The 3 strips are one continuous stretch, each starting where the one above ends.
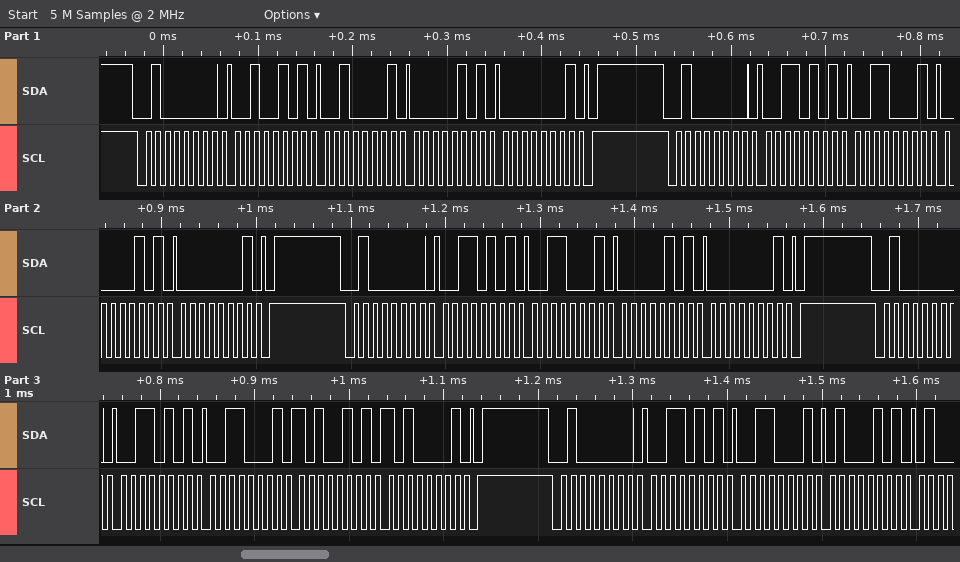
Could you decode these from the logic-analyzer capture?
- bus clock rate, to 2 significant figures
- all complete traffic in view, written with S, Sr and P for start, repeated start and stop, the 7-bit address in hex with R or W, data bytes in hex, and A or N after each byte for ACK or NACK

100 kHz
S 20W A 25 A 21 A 05 A 01 A P S 20W A 35 A 31 A 05 A 01 A P S 20W A 35 A 31 A 05 A 01 A P S 20W A 35 A 31 A A5 A A1 A P S 20W A 35 A 31 A 45 A
